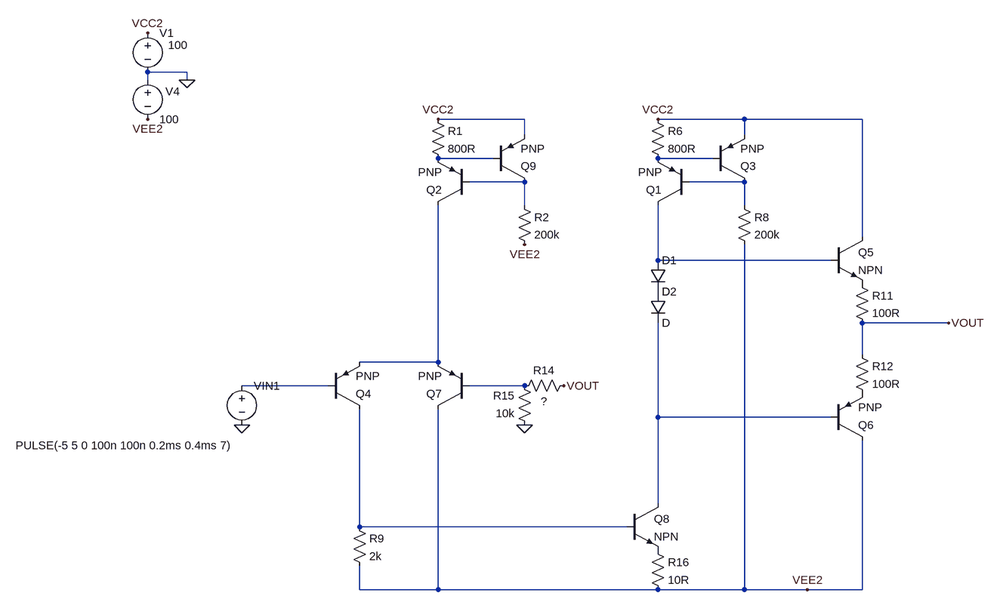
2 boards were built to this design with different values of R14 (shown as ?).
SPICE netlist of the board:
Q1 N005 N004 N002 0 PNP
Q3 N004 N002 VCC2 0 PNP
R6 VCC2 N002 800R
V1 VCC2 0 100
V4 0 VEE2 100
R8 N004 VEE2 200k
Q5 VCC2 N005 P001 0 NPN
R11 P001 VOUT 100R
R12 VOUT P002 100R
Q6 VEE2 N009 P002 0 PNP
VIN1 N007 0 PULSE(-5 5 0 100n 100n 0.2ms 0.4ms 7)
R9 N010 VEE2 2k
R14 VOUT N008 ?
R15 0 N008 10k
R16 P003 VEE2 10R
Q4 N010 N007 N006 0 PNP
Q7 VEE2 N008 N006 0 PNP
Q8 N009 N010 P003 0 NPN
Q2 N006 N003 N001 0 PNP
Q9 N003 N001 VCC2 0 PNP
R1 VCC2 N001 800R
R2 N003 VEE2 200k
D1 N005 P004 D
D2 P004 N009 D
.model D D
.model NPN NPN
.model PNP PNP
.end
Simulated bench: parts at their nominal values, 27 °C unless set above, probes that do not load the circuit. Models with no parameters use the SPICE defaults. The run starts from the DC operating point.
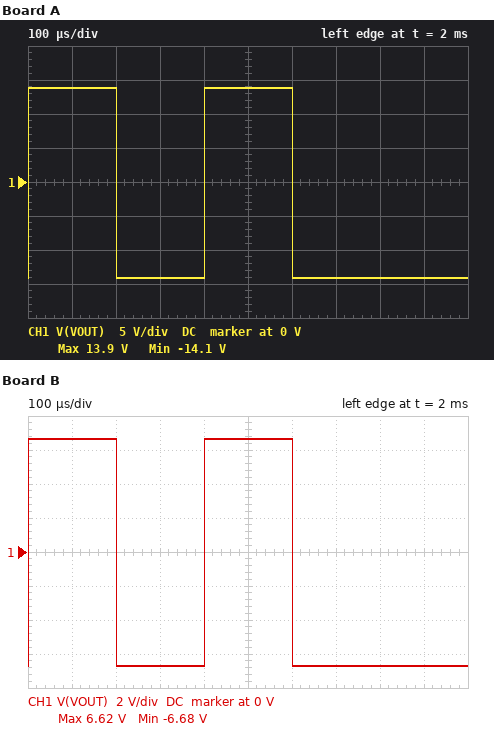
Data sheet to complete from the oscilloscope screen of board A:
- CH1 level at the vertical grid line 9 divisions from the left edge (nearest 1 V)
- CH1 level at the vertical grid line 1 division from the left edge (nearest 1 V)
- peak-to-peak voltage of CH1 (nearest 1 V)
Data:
-14 V
14 V
28 V
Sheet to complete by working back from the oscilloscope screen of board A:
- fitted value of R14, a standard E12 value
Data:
18 kΩ
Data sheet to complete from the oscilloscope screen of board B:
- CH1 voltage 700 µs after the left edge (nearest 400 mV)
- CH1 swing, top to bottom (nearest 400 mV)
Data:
-6.8 V
13.2 V
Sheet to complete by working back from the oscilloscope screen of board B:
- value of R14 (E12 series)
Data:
3.3 kΩ
